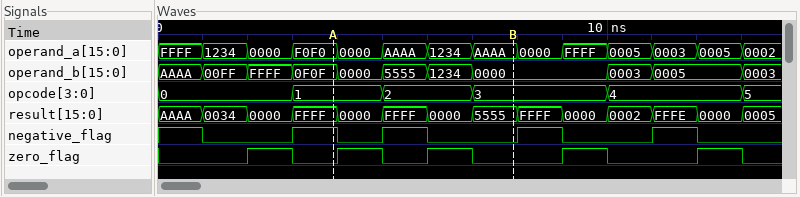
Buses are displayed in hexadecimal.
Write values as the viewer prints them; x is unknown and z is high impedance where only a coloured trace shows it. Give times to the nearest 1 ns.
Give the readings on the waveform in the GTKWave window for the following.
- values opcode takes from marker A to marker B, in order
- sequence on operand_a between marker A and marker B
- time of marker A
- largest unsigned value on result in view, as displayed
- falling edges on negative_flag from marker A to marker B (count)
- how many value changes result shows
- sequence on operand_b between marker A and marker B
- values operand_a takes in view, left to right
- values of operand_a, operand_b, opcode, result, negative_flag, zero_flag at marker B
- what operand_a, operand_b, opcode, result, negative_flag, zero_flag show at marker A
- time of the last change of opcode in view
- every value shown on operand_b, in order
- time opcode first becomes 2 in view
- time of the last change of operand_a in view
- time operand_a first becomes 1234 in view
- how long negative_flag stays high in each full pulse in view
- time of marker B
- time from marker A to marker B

1, 2, 3
F0F0, 0000, AAAA, 1234, AAAA
4 ns
FFFF
2
13
0F0F, 0000, 5555, 1234, 0000
FFFF, 1234, 0000, F0F0, 0000, AAAA, 1234, AAAA, 0000, FFFF, 0005, 0003, 0005, 0002
operand_a=AAAA, operand_b=0000, opcode=3, result=5555, negative_flag=0, zero_flag=0
operand_a=F0F0, operand_b=0F0F, opcode=1, result=FFFF, negative_flag=1, zero_flag=0
13 ns
AAAA, 00FF, FFFF, 0F0F, 0000, 5555, 1234, 0000, 0003, 0005, 0003
5 ns
13 ns
1 ns
1 ns, 1 ns, 1 ns, 1 ns
8 ns
4 ns
